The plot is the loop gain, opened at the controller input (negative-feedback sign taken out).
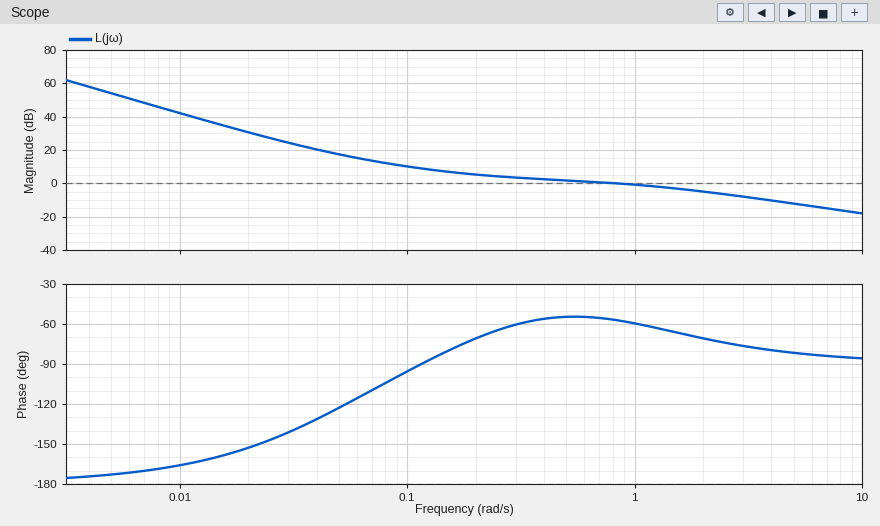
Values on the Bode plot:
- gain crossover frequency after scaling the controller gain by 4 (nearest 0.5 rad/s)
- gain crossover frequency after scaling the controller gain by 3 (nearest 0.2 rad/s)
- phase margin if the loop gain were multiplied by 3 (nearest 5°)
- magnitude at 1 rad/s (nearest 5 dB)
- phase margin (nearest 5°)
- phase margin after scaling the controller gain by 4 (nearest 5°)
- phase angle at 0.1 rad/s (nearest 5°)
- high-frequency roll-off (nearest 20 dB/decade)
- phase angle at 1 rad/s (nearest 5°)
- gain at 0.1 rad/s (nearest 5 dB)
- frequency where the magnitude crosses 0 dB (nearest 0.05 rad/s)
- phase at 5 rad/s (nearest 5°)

5.0 rad/s
3.6 rad/s
100°
0 dB
125°
100°
-95°
-20 dB/decade
-60°
10 dB
0.85 rad/s
-80°
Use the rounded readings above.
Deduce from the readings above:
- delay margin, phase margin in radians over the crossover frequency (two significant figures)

2.6 s
